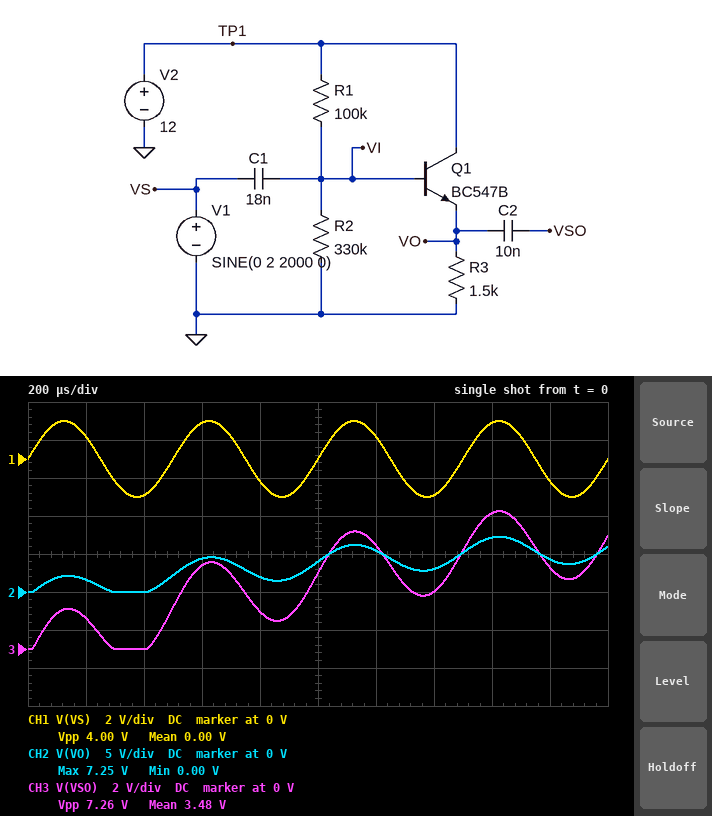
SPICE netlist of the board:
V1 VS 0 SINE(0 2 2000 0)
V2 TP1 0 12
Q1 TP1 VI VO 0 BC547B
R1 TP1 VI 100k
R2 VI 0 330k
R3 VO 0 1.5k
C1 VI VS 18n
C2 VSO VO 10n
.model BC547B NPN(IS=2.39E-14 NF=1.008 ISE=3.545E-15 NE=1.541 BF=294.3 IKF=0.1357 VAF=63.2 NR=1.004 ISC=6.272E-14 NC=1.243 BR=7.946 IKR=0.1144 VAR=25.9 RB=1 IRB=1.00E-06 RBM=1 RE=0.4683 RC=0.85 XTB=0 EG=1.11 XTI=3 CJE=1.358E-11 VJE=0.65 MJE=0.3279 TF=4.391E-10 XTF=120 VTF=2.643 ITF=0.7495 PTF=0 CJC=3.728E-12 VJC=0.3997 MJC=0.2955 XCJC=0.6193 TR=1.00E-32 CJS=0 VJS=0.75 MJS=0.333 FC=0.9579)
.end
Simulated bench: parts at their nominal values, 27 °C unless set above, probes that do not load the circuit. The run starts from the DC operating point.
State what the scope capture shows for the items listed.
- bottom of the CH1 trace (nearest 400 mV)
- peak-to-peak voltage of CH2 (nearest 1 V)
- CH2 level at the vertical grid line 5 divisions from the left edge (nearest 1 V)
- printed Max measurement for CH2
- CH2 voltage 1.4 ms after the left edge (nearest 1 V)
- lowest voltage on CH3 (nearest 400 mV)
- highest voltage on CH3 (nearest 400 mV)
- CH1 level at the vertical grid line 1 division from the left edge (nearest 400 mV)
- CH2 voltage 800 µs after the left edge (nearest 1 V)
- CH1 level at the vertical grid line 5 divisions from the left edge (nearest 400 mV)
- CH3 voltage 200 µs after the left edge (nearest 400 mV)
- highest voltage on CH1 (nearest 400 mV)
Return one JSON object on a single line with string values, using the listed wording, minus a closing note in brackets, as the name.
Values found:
{"bottom of the CH1 trace": "-2.0 V", "peak-to-peak voltage of CH2": "7 V", "CH2 level at the vertical grid line 5 divisions from the left edge": "4 V", "printed Max measurement for CH2": "7.25 V", "CH2 voltage 1.4 ms after the left edge": "3 V", "lowest voltage on CH3": "0 V", "highest voltage on CH3": "7.2 V", "CH1 level at the vertical grid line 1 division from the left edge": "1.2 V", "CH2 voltage 800 µs after the left edge": "2 V", "CH1 level at the vertical grid line 5 divisions from the left edge": "0 V", "CH3 voltage 200 µs after the left edge": "1.6 V", "highest voltage on CH1": "2.0 V"}
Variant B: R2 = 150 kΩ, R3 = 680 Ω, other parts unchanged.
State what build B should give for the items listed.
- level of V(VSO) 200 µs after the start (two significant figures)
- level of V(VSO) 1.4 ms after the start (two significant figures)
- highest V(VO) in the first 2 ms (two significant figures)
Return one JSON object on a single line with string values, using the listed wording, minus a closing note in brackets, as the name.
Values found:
{"level of V(VSO) 200 µs after the start": "1.5 V", "level of V(VSO) 1.4 ms after the start": "2.1 V", "highest V(VO) in the first 2 ms": "6.2 V"}
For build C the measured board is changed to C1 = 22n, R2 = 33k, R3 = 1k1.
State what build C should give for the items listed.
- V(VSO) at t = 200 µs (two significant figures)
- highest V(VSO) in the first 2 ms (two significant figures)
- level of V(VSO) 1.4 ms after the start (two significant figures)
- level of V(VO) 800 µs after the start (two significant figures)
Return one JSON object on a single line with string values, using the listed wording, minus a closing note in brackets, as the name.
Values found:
{"V(VSO) at t = 200 µs": "1.0 V", "highest V(VSO) in the first 2 ms": "4.0 V", "level of V(VSO) 1.4 ms after the start": "260 mV", "level of V(VO) 800 µs after the start": "190 mV"}
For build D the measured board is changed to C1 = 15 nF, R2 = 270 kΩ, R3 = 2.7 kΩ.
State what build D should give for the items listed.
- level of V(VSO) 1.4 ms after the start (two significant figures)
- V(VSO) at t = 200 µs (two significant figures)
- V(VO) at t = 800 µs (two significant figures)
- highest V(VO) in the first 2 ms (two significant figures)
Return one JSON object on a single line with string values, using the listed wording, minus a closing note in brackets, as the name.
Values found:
{"level of V(VSO) 1.4 ms after the start": "3.6 V", "V(VSO) at t = 200 µs": "1.8 V", "V(VO) at t = 800 µs": "2.5 V", "highest V(VO) in the first 2 ms": "7.8 V"}
